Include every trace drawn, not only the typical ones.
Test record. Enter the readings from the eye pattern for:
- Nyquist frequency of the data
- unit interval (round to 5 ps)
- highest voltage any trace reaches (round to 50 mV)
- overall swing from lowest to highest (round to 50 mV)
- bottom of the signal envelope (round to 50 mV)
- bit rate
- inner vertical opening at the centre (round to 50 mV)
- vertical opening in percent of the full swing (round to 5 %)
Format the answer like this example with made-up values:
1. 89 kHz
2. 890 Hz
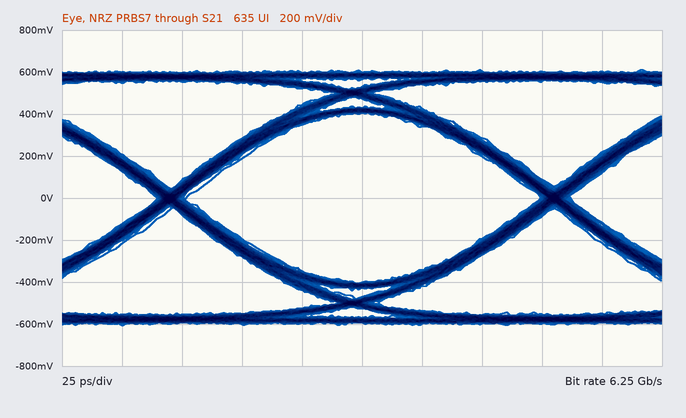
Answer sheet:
1. 3.125 GHz
2. 160 ps
3. 600 mV
4. 1.20 V
5. -600 mV
6. 6.25 Gb/s
7. 800 mV
8. 65 %
